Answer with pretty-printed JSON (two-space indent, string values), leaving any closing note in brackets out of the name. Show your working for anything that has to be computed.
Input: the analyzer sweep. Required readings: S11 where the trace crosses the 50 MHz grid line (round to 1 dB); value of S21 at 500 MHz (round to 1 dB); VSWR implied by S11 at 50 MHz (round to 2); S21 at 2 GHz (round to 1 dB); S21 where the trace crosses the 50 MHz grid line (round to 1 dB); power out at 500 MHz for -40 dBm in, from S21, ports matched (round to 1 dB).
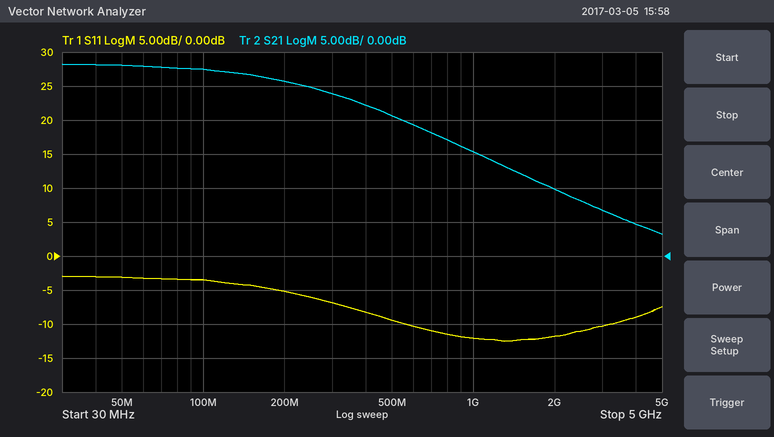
{
  "S11 where the trace crosses the 50 MHz grid line": "-3 dB",
  "value of S21 at 500 MHz": "21 dB",
  "VSWR implied by S11 at 50 MHz": "|Γ| = 10^(-3/20) = 0.7079; VSWR = (1 + 0.7079)/(1 − 0.7079) ≈ 6",
  "S21 at 2 GHz": "10 dB",
  "S21 where the trace crosses the 50 MHz grid line": "28 dB",
  "power out at 500 MHz for -40 dBm in, from S21, ports matched": "-40 dBm + (21 dB) = -19 dBm"
}
